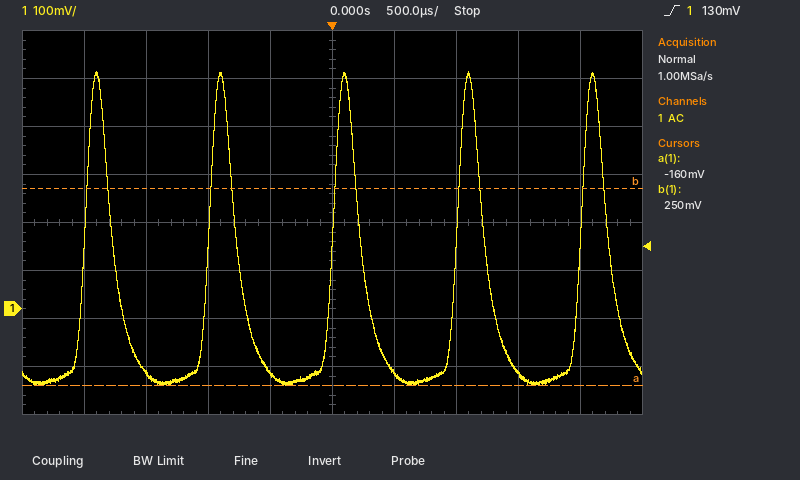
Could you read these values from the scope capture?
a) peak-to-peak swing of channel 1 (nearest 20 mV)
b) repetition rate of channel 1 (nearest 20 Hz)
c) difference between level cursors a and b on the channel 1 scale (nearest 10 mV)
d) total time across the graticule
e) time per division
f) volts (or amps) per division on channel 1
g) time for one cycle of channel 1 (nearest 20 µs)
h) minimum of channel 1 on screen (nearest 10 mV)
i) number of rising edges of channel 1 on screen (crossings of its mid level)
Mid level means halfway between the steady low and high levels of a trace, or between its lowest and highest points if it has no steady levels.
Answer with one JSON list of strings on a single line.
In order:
["660 mV", "1.00 kHz", "410 mV", "5 ms", "500 µs", "100 mV", "1.00 ms", "-160 mV", "5"]
